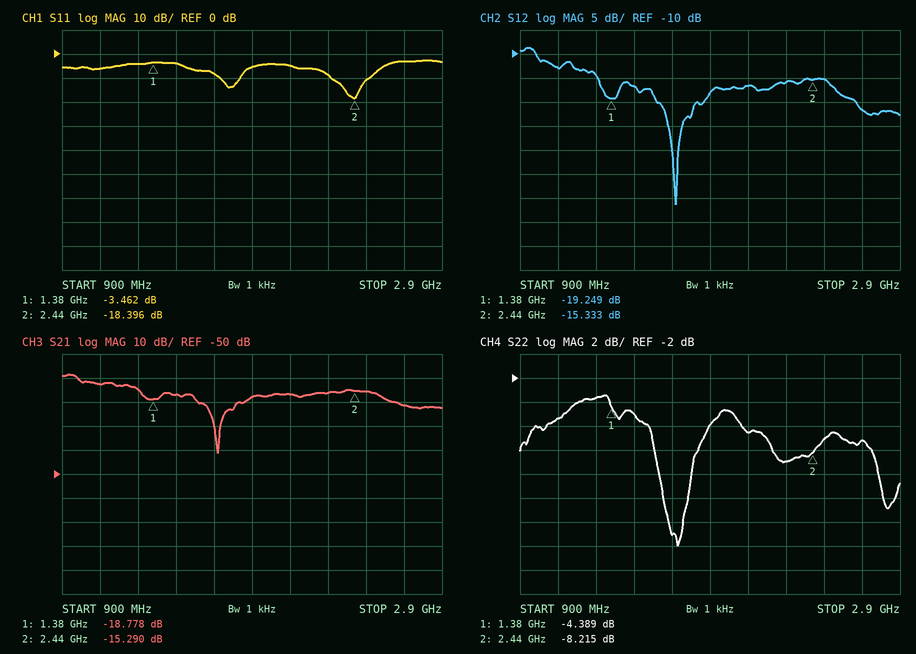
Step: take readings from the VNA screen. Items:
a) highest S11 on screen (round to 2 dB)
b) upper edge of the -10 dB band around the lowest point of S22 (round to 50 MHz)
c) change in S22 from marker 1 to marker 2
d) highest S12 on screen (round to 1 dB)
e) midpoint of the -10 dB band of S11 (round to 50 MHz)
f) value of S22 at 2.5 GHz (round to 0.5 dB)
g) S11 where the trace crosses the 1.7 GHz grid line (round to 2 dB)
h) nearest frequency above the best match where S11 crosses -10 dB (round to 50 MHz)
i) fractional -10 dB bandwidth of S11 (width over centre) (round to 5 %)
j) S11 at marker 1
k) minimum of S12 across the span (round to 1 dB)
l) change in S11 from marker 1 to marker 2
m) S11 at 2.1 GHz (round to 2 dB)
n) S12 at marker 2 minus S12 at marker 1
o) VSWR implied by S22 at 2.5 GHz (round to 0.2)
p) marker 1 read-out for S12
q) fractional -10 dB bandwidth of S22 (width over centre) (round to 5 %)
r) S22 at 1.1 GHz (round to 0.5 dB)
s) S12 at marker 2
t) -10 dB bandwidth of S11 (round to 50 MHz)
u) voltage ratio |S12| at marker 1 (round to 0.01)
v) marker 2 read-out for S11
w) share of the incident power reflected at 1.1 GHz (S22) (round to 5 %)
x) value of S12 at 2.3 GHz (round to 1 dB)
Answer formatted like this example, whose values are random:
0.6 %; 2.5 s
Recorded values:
-2 dB; 1.80 GHz; -3.826 dB; -9 dB; 2.40 GHz; -7.0 dB; -8 dB; 2.50 GHz; 10 %; -3.462 dB; -41 dB; -14.934 dB; -4 dB; 3.916 dB; 2.6; -19.249 dB; 10 %; -5.5 dB; -15.333 dB; 200 MHz; 0.11; -18.396 dB; 30 %; -16 dB
